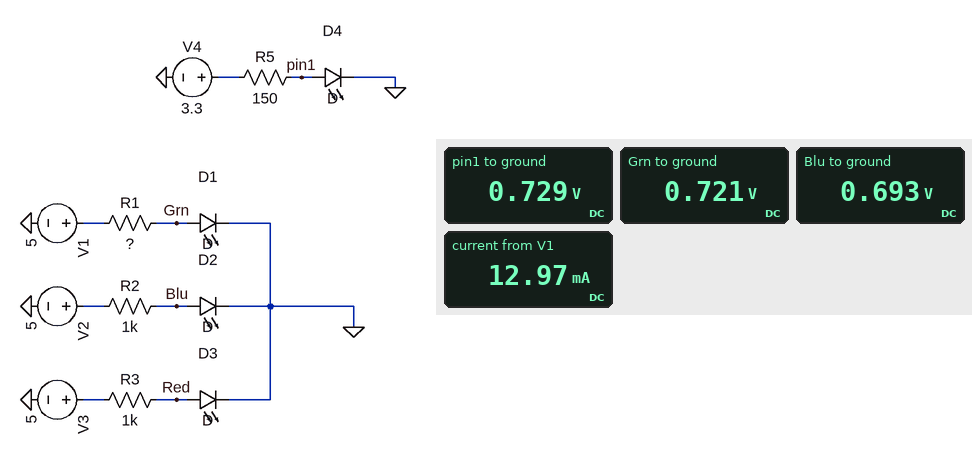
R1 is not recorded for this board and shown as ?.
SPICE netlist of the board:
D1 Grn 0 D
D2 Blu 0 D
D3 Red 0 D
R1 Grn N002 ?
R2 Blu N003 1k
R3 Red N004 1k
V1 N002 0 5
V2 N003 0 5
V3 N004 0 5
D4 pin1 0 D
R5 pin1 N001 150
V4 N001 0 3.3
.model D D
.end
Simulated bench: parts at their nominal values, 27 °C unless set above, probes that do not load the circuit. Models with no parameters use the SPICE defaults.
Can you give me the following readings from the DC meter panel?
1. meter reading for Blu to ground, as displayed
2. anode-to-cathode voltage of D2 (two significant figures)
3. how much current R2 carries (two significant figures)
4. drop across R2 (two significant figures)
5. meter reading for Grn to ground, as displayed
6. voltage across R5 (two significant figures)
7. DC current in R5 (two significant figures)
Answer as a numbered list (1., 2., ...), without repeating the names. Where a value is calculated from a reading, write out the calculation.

1. 0.693 V
2. 693 mV = 690 mV
3. (5 V - 693 mV) / 1 kΩ = 4.3 mA
4. 5 V - 693 mV = 4.3 V
5. 0.721 V
6. 3.3 V - 729 mV = 2.6 V
7. (3.3 V - 729 mV) / 150 Ω = 17 mA
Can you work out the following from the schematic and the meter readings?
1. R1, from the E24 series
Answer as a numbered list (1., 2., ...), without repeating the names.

1. 330 Ω
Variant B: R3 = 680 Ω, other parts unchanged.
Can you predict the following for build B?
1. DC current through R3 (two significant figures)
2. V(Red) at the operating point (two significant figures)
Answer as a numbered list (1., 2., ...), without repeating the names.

1. 6.3 mA
2. 700 mV
